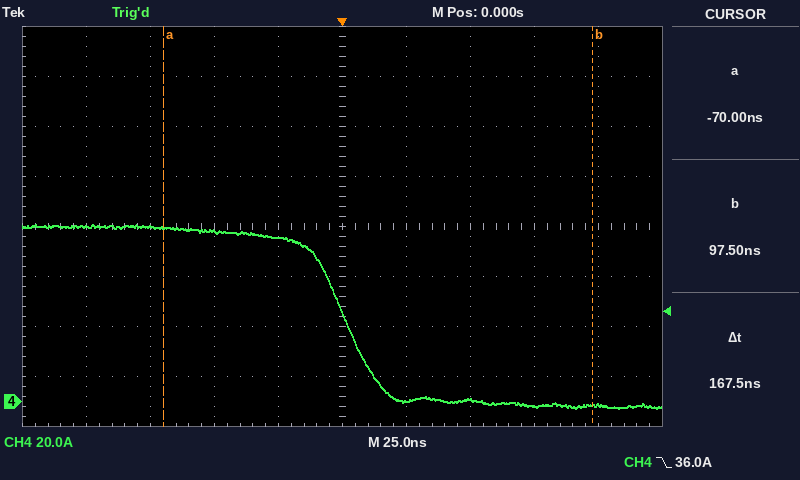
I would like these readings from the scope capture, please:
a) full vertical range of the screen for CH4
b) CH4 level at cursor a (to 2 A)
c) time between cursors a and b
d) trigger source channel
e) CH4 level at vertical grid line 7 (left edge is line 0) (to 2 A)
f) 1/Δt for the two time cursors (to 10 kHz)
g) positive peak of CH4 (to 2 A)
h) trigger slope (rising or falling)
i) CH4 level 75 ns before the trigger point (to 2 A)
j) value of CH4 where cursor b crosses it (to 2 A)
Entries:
160 A
70 A
167.5 ns
CH4
0 A
5.97 MHz
70 A
falling
70 A
-2 A
